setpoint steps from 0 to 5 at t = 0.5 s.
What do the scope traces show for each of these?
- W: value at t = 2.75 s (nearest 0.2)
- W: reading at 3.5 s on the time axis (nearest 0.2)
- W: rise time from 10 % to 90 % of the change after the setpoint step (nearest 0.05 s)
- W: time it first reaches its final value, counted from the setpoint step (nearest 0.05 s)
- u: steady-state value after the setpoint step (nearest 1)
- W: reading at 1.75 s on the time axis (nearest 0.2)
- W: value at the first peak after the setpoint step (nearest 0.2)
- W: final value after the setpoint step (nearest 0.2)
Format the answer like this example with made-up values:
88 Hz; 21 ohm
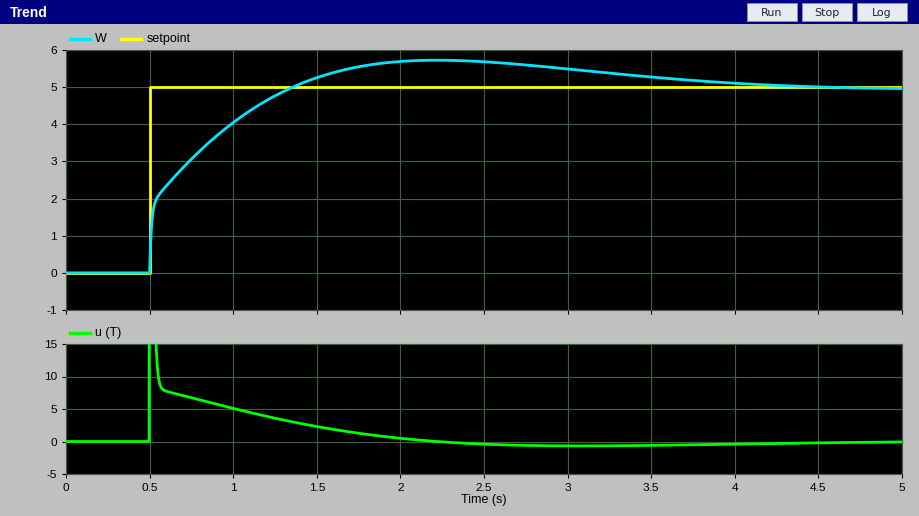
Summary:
5.6; 5.2; 0.65 s; 0.85 s; 0; 5.6; 5.8; 5.0
